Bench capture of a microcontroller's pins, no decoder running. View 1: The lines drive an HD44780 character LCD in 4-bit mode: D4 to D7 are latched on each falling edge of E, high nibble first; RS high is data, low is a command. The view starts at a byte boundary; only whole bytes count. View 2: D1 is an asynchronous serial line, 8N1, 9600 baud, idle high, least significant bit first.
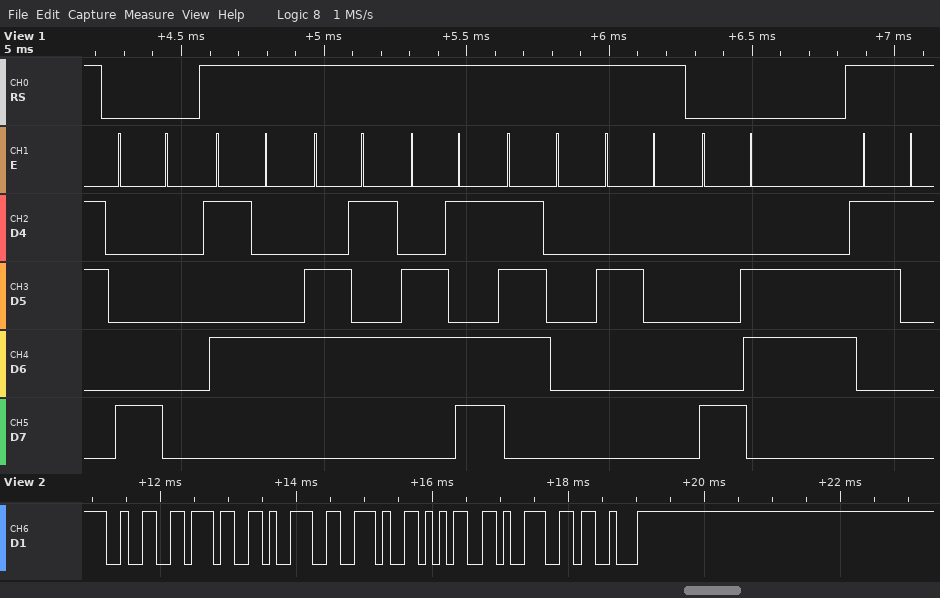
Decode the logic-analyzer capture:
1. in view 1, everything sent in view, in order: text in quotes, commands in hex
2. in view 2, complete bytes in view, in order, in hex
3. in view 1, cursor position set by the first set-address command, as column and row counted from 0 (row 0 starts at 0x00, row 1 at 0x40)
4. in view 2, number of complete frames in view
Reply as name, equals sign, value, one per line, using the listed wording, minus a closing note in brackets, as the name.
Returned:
in view 1, everything sent in view, in order: text in quotes, commands in hex = 0x80 "Temp " 0x86 "1"
in view 2, complete bytes in view, in order, in hex = 32 37 39 2E 35 39 13
in view 1, cursor position set by the first set-address command, as column and row counted from 0 = column 0, row 0
in view 2, number of complete frames in view = 7
